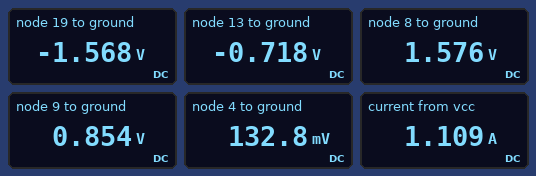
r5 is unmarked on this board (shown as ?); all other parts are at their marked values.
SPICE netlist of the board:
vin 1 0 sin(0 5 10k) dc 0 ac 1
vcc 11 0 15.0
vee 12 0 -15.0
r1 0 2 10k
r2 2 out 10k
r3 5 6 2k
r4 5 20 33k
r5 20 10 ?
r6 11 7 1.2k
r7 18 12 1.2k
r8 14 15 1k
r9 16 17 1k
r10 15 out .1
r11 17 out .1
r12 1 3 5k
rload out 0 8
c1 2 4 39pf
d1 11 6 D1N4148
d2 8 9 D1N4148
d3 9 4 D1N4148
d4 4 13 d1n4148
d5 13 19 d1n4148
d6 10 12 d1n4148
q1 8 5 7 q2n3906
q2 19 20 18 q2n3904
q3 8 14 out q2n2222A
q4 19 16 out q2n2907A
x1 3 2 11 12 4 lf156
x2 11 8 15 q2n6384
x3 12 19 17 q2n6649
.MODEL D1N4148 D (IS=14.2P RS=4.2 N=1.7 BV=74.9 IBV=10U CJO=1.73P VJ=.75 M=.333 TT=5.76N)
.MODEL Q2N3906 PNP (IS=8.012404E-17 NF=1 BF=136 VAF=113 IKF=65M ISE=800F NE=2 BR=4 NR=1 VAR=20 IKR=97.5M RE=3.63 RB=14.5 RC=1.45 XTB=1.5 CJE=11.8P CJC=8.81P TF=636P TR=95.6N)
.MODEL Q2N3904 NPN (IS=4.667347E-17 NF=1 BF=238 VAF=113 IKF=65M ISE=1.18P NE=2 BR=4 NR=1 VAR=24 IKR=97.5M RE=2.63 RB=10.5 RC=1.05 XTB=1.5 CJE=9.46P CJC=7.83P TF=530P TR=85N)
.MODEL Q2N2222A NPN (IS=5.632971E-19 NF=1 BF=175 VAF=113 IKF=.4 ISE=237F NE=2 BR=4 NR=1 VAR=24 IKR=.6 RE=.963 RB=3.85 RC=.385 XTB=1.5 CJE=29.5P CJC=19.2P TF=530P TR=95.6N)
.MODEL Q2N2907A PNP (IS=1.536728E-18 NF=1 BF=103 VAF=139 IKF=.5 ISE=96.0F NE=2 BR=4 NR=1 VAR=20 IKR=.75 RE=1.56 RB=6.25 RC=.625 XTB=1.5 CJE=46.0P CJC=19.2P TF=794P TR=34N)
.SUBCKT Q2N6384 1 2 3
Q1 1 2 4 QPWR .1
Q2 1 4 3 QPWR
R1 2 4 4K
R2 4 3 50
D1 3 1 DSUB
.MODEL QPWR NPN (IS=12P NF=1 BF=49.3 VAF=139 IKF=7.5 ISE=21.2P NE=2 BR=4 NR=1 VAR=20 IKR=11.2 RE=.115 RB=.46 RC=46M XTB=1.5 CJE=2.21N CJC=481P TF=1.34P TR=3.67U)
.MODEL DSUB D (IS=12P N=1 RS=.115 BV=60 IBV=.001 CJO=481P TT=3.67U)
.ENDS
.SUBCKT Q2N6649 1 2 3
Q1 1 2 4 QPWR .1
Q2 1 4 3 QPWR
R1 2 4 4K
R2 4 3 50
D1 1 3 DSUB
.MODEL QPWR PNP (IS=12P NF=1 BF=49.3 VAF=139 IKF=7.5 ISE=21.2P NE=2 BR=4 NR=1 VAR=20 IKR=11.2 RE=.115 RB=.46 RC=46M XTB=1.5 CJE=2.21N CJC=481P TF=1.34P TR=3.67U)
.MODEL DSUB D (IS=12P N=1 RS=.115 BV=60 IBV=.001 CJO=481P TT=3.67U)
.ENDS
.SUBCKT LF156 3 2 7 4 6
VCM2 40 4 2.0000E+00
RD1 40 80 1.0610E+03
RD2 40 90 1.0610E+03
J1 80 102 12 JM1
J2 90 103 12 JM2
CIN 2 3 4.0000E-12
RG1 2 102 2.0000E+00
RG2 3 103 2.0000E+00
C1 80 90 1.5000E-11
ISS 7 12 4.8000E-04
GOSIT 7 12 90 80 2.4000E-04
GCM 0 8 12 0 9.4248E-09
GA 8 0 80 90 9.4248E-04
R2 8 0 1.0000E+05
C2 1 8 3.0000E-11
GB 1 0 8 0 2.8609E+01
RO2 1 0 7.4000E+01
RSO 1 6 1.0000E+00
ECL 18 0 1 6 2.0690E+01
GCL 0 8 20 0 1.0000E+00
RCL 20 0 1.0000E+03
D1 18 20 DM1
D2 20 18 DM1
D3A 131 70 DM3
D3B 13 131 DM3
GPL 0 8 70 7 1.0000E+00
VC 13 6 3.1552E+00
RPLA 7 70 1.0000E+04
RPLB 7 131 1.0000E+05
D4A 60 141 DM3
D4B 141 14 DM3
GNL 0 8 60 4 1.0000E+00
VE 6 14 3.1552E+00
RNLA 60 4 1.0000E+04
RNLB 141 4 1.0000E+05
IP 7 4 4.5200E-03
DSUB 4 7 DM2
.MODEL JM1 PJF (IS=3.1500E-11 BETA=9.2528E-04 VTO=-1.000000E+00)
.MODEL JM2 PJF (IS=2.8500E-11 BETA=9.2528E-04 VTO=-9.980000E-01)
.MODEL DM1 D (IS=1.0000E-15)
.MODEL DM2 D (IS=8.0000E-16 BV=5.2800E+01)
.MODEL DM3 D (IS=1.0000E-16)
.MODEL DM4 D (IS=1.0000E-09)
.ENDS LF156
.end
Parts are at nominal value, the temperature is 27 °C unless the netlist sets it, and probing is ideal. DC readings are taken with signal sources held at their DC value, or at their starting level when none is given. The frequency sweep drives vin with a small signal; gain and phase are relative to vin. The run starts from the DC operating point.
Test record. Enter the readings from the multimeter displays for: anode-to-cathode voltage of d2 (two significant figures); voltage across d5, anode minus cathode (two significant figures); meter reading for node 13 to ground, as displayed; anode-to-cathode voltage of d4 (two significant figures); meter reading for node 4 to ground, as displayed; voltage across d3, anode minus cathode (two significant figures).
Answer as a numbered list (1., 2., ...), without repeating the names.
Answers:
1. 720 mV
2. 850 mV
3. -0.718 V
4. 850 mV
5. 132.8 mV
6. 720 mV
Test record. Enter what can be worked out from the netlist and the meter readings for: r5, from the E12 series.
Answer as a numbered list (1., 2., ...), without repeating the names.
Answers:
1. 6.8 kΩ
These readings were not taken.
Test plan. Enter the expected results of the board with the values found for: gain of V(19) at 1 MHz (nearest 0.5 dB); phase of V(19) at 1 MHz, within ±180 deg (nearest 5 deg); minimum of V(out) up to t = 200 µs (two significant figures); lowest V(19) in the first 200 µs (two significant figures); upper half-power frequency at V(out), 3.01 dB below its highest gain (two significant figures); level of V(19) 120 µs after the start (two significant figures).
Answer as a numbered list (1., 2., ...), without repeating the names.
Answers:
1. 1.5 dB
2. -35 deg
3. -10 V
4. -12 V
5. 510 kHz
6. 8.3 V
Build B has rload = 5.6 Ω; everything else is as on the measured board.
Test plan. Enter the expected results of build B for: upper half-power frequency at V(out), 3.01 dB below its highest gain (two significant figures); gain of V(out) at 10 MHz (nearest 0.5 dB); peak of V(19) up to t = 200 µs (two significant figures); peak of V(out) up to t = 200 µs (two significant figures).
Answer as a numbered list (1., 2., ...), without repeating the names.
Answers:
1. 500 kHz
2. -18.5 dB
3. 11 V
4. 7.3 V
